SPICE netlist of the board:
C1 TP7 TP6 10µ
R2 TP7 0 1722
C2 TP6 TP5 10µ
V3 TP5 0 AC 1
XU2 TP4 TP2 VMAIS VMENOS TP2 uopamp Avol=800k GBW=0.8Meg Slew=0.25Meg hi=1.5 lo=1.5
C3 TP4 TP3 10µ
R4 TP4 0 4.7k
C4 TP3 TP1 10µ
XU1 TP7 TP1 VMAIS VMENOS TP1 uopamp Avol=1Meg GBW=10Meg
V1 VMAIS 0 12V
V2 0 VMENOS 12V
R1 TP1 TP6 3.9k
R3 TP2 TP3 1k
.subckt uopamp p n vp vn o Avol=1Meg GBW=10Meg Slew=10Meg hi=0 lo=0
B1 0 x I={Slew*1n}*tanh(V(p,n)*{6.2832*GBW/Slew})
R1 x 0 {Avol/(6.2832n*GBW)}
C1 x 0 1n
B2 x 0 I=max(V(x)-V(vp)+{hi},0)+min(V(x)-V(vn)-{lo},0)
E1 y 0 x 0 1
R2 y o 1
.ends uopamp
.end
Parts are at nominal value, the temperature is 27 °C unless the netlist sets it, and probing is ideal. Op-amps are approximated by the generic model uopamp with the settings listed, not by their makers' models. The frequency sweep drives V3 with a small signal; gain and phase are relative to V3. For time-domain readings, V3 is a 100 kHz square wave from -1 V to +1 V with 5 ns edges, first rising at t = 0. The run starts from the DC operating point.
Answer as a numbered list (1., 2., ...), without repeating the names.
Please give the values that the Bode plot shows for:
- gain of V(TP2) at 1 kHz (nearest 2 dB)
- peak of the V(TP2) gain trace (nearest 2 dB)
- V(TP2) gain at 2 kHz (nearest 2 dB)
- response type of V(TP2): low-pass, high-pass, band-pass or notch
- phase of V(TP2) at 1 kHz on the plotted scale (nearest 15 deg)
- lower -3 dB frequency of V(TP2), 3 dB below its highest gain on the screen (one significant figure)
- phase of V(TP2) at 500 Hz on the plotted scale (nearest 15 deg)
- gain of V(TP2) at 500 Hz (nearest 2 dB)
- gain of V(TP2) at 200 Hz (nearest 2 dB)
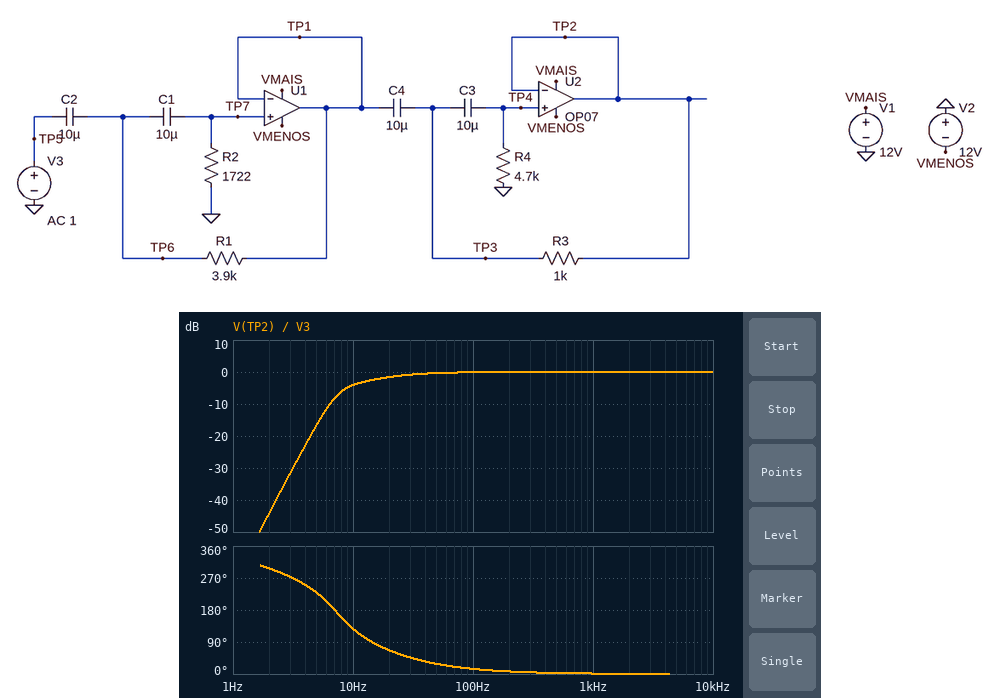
1. 0 dB
2. 0 dB
3. 0 dB
4. high-pass
5. 0 deg
6. 10 Hz
7. 0 deg
8. 0 dB
9. 0 dB
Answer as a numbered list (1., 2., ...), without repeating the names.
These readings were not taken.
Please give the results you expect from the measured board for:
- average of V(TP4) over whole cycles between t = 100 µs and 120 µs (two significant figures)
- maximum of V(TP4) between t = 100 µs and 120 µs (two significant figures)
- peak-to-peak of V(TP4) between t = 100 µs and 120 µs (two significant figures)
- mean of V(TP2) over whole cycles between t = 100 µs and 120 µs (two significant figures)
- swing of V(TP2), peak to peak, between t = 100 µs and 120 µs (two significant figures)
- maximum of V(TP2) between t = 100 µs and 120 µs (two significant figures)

1. 980 mV
2. 2.0 V
3. 2.0 V
4. 870 mV
5. 1.3 V
6. 1.5 V
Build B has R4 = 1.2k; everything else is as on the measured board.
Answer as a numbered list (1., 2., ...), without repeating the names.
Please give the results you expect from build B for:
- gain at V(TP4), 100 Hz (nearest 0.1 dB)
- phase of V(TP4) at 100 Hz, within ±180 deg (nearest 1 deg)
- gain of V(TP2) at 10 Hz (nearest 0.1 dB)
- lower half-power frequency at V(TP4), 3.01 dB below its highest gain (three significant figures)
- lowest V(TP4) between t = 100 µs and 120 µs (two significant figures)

1. -0.2 dB
2. 26 deg
3. -15.0 dB
4. 27.1 Hz
5. -36 mV
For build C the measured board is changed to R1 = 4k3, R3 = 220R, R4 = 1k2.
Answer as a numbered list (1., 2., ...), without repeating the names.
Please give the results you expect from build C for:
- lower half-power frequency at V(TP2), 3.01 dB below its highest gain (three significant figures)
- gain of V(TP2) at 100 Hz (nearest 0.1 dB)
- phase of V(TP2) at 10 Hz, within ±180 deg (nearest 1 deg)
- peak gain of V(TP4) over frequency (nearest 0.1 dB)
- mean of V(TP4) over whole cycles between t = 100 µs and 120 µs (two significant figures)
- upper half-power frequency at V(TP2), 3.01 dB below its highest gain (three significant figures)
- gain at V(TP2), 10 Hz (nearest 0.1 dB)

1. 27.3 Hz
2. 0.4 dB
3. -127 deg
4. 1.5 dB
5. 960 mV
6. 503 kHz
7. -24.9 dB
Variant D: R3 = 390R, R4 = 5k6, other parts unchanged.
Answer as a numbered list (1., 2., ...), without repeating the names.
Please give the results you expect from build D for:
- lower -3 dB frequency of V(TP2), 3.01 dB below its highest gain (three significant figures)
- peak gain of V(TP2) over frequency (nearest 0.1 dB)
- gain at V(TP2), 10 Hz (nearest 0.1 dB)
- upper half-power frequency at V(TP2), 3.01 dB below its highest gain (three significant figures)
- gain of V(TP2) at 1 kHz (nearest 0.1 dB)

1. 9.78 Hz
2. 1.2 dB
3. -1.2 dB
4. 567 kHz
5. 0 dB
